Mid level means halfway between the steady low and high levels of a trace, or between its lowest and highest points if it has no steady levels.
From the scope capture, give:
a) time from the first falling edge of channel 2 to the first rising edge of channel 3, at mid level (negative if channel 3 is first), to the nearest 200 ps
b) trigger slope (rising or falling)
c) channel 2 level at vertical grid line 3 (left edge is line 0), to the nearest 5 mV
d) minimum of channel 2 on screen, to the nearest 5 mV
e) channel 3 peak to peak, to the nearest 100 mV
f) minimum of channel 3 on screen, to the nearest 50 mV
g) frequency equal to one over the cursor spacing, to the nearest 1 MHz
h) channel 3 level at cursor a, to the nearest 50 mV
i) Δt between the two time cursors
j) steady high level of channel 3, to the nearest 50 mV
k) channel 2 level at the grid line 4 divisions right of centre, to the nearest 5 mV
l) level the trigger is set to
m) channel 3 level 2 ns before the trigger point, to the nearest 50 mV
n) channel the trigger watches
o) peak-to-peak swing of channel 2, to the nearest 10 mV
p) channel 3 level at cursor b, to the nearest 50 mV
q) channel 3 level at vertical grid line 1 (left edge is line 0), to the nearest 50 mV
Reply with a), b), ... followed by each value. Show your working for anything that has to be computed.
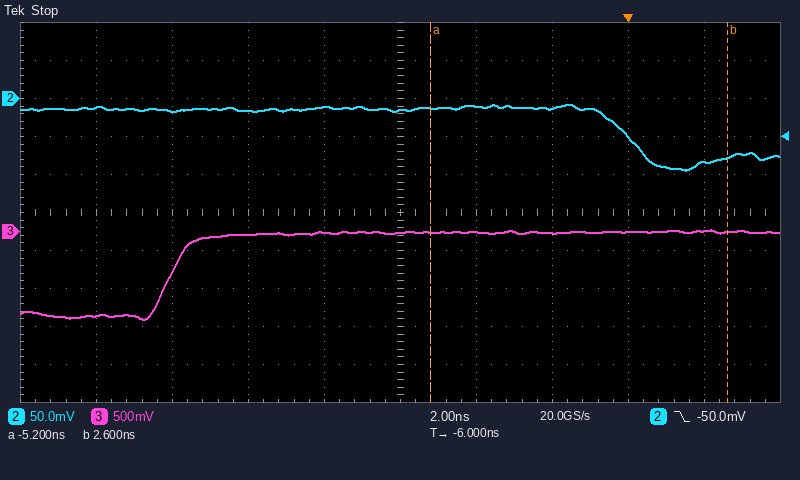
a) -12.0 ns
b) falling
c) -15 mV
d) -95 mV
e) 1.20 V
f) -1.15 V
g) 1 / 7.8 ns ≈ 128 MHz
h) 0 mV
i) 2.6 ns − (-5.2 ns) = 7.8 ns
j) 0 mV
k) -85 mV
l) -50.0 mV
m) 0 mV
n) channel 2
o) 90 mV
p) 0 mV
q) -1.10 V
